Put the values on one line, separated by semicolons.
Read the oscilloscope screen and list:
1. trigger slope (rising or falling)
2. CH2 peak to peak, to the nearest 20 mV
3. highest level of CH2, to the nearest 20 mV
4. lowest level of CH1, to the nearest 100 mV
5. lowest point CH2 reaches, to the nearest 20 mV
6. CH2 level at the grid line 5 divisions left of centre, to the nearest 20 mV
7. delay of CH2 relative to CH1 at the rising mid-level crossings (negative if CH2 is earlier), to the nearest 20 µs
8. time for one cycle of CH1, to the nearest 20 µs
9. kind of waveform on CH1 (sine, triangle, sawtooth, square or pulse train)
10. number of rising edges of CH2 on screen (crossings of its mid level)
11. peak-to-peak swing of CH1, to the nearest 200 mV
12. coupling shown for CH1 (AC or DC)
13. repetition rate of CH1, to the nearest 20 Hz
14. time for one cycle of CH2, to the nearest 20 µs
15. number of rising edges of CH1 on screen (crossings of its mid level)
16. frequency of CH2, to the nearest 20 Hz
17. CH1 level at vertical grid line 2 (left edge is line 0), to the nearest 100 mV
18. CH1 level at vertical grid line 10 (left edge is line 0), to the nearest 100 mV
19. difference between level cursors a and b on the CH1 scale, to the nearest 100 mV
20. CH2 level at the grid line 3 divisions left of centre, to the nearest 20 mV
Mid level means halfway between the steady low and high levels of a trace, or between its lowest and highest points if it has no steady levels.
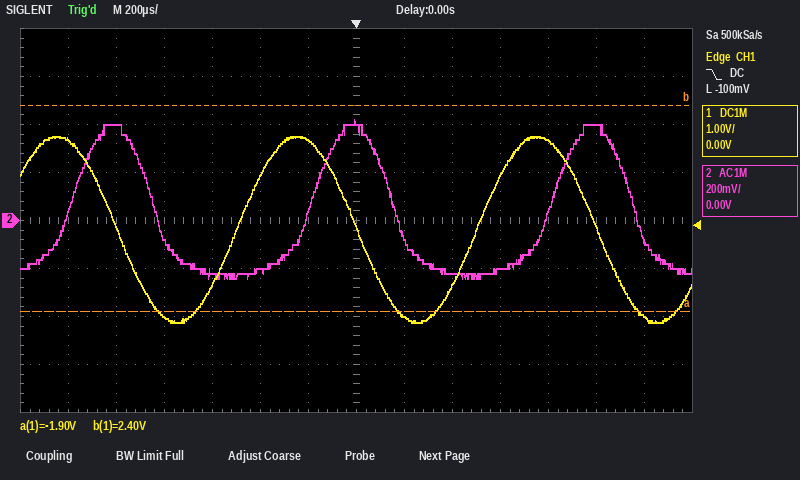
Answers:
falling; 660 mV; 420 mV; -2.1 V; -240 mV; 400 mV; +320 µs; 1.00 ms; sine; 3; 3.8 V; DC; 1.00 kHz; 1.00 ms; 2; 1.00 kHz; -100 mV; 900 mV; 4.3 V; -220 mV
